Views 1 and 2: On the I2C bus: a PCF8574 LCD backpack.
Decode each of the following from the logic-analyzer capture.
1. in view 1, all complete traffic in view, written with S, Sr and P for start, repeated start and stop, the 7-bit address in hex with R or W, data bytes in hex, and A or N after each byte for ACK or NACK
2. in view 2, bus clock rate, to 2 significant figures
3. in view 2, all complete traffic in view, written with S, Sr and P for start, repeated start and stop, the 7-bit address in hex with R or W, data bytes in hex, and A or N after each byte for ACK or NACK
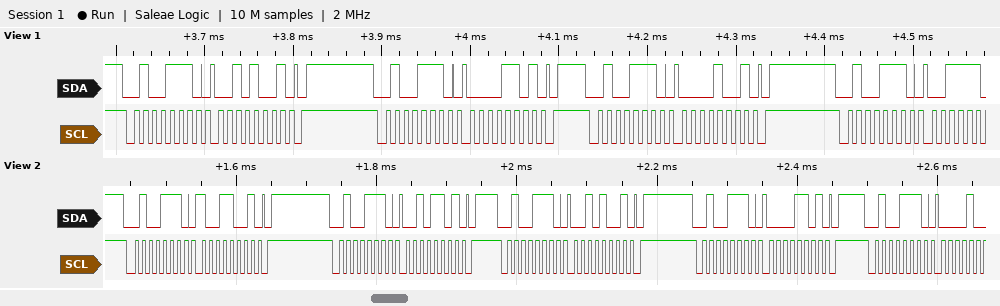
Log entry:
S 27W A 29 A P S 27W A 0D A P S 27W A 09 A P S 27W A
100 kHz
S 27W A 99 A P S 27W A 2D A P S 27W A 29 A P S 27W A 0D A P S 27W A
